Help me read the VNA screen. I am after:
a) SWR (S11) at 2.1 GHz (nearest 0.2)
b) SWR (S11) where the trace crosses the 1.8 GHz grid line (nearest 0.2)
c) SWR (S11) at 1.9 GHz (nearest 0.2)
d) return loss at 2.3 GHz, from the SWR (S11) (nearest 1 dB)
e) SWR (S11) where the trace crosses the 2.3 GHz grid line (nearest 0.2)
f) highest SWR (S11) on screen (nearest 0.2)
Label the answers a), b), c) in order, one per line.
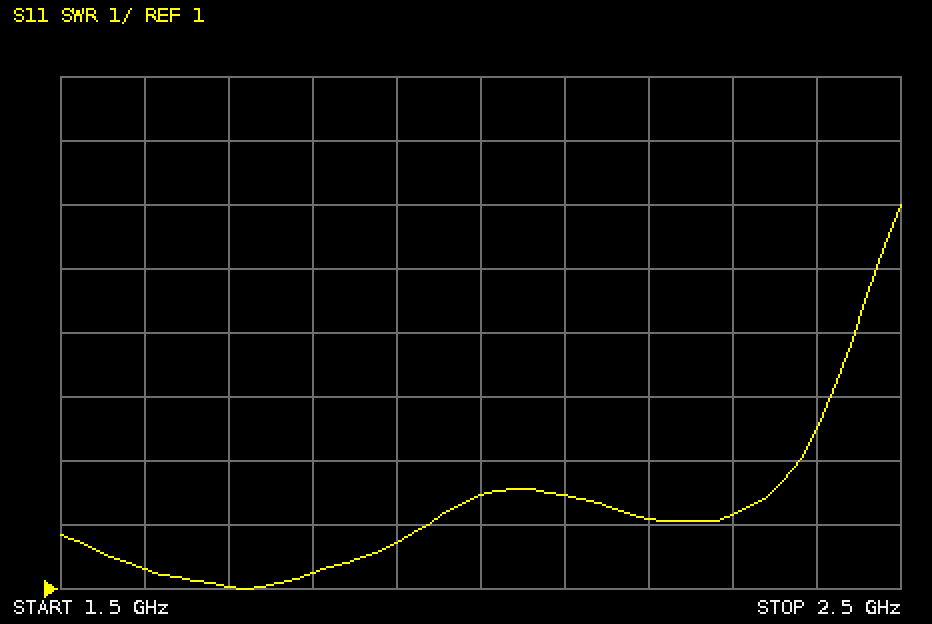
a) 2.4
b) 1.2
c) 1.8
d) 9 dB
e) 2.2
f) 7.0
